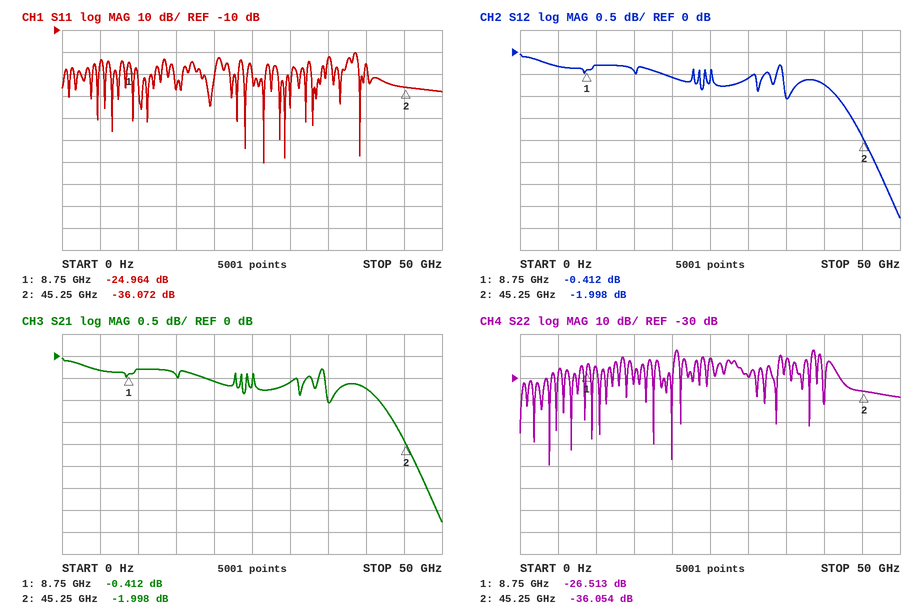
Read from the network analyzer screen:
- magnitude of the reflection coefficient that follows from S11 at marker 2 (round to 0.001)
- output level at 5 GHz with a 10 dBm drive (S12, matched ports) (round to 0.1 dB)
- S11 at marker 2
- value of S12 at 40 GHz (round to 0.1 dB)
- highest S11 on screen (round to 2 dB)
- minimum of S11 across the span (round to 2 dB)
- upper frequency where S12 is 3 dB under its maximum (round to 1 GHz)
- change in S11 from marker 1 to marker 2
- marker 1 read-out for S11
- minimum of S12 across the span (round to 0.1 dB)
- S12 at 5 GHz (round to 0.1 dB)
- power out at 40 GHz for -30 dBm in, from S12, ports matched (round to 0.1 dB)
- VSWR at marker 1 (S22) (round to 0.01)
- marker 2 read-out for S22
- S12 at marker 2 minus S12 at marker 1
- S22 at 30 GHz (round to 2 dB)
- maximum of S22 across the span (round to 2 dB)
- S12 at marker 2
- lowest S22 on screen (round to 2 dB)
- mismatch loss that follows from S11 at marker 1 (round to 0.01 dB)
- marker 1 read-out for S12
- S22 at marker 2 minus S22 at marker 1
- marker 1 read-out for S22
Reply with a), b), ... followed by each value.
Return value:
a) 0.016
b) 9.7 dBm
c) -36.072 dB
d) -0.7 dB
e) -20 dB
f) -70 dB
g) 48 GHz
h) -11.108 dB
i) -24.964 dB
j) -3.8 dB
k) -0.3 dB
l) -30.7 dBm
m) 1.10
n) -36.054 dB
o) -1.586 dB
p) -30 dB
q) -18 dB
r) -1.998 dB
s) -70 dB
t) 0.01 dB
u) -0.412 dB
v) -9.541 dB
w) -26.513 dB
